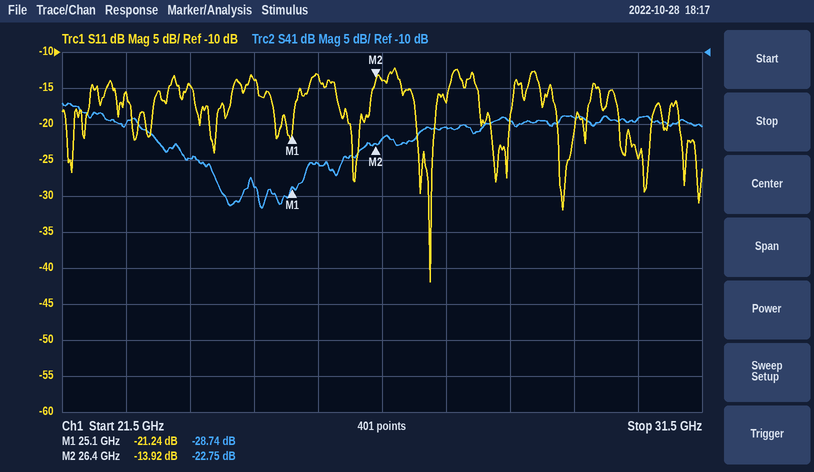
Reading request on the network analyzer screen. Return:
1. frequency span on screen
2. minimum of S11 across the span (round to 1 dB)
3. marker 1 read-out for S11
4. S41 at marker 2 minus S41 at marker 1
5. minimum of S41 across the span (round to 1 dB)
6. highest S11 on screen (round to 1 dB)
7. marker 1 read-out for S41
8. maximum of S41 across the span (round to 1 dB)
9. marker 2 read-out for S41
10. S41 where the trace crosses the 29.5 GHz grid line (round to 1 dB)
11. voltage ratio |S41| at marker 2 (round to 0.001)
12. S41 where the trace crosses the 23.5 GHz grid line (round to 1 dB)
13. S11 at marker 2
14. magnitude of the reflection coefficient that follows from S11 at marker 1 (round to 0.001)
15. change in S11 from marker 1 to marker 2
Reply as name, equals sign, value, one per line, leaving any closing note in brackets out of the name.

frequency span on screen = 10 GHz
minimum of S11 across the span = -42 dB
marker 1 read-out for S11 = -21.24 dB
S41 at marker 2 minus S41 at marker 1 = 5.99 dB
minimum of S41 across the span = -32 dB
highest S11 on screen = -12 dB
marker 1 read-out for S41 = -28.74 dB
maximum of S41 across the span = -17 dB
marker 2 read-out for S41 = -22.75 dB
S41 where the trace crosses the 29.5 GHz grid line = -19 dB
voltage ratio |S41| at marker 2 = 0.073
S41 where the trace crosses the 23.5 GHz grid line = -25 dB
S11 at marker 2 = -13.92 dB
magnitude of the reflection coefficient that follows from S11 at marker 1 = 0.087
change in S11 from marker 1 to marker 2 = 7.32 dB
